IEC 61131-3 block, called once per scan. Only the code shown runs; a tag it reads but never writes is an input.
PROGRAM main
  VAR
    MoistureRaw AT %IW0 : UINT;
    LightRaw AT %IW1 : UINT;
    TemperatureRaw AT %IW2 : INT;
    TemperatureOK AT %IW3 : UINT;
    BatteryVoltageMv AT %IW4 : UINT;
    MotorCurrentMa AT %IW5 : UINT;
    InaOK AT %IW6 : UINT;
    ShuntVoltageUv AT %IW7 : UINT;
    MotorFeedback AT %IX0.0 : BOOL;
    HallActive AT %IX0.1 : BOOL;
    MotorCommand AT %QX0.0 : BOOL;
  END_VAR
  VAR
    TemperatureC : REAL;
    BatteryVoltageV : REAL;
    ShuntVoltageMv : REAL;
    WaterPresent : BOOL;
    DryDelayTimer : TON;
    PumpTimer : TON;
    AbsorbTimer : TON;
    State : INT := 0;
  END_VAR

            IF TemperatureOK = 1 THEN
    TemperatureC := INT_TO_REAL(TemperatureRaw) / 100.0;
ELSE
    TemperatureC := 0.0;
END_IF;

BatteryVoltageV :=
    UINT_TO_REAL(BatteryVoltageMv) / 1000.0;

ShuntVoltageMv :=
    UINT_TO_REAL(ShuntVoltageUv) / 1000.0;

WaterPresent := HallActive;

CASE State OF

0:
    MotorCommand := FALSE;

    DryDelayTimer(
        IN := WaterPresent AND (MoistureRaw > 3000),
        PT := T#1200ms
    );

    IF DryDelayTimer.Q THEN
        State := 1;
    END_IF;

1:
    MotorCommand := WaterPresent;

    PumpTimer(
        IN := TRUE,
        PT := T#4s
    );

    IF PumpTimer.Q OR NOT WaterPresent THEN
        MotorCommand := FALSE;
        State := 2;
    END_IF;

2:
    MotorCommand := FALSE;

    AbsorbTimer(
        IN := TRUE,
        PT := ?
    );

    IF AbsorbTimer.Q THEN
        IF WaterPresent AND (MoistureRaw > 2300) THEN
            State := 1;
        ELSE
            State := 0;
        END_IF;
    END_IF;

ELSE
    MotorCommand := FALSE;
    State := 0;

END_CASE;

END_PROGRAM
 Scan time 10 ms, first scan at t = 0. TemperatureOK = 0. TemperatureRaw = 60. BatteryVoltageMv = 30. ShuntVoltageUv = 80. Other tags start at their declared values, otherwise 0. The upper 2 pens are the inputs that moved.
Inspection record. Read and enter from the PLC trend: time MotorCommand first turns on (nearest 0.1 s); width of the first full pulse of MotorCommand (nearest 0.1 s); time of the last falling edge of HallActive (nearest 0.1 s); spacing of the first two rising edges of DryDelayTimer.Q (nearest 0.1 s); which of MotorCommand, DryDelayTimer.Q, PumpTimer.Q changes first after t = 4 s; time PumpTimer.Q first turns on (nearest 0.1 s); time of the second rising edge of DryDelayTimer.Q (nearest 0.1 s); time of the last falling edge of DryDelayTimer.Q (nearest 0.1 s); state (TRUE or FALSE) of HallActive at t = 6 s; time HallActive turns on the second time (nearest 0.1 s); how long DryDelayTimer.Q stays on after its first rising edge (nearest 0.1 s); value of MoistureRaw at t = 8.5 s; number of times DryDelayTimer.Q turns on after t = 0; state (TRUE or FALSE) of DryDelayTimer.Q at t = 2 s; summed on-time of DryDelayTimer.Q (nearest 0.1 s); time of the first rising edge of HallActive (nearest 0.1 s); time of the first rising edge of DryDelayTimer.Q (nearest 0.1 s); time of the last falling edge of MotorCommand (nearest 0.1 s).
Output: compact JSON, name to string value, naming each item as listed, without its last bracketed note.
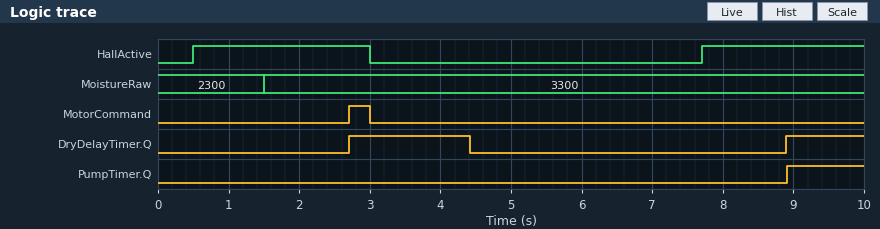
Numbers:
{"time MotorCommand first turns on": "2.7 s", "width of the first full pulse of MotorCommand": "0.3 s", "time of the last falling edge of HallActive": "3.0 s", "spacing of the first two rising edges of DryDelayTimer.Q": "6.2 s", "which of MotorCommand, DryDelayTimer.Q, PumpTimer.Q changes first after t = 4 s": "DryDelayTimer.Q", "time PumpTimer.Q first turns on": "8.9 s", "time of the second rising edge of DryDelayTimer.Q": "8.9 s", "time of the last falling edge of DryDelayTimer.Q": "4.4 s", "state (TRUE or FALSE) of HallActive at t = 6 s": "FALSE", "time HallActive turns on the second time": "7.7 s", "how long DryDelayTimer.Q stays on after its first rising edge": "1.7 s", "value of MoistureRaw at t = 8.5 s": "3300", "number of times DryDelayTimer.Q turns on after t = 0": "2", "state (TRUE or FALSE) of DryDelayTimer.Q at t = 2 s": "FALSE", "summed on-time of DryDelayTimer.Q": "2.8 s", "time of the first rising edge of HallActive": "0.5 s", "time of the first rising edge of DryDelayTimer.Q": "2.7 s", "time of the last falling edge of MotorCommand": "3.0 s"}
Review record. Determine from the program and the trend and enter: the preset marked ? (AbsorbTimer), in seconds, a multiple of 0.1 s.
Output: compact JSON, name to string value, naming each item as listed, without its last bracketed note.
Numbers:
{"the preset marked ? (AbsorbTimer), in seconds, a multiple of 0.1 s": "1.4 s"}
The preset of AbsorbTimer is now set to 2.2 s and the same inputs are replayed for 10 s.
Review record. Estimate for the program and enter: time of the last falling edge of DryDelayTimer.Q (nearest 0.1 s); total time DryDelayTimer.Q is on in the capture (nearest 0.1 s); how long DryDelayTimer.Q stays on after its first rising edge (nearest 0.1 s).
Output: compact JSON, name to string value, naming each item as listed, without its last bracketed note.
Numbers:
{"time of the last falling edge of DryDelayTimer.Q": "5.2 s", "total time DryDelayTimer.Q is on in the capture": "3.6 s", "how long DryDelayTimer.Q stays on after its first rising edge": "2.5 s"}
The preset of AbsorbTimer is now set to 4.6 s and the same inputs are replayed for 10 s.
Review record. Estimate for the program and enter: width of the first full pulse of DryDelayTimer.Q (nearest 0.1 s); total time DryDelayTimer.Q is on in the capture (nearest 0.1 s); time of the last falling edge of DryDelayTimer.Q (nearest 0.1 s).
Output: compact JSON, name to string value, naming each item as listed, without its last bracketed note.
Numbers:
{"width of the first full pulse of DryDelayTimer.Q": "4.9 s", "total time DryDelayTimer.Q is on in the capture": "6.0 s", "time of the last falling edge of DryDelayTimer.Q": "7.6 s"}
